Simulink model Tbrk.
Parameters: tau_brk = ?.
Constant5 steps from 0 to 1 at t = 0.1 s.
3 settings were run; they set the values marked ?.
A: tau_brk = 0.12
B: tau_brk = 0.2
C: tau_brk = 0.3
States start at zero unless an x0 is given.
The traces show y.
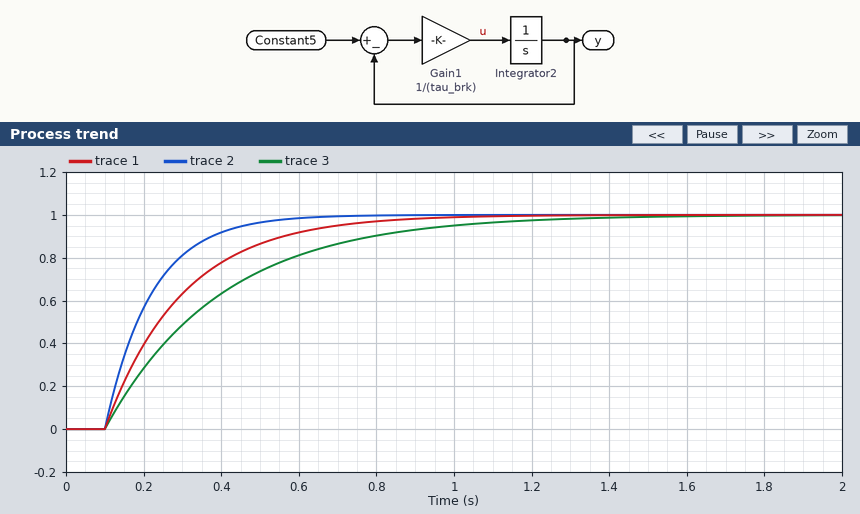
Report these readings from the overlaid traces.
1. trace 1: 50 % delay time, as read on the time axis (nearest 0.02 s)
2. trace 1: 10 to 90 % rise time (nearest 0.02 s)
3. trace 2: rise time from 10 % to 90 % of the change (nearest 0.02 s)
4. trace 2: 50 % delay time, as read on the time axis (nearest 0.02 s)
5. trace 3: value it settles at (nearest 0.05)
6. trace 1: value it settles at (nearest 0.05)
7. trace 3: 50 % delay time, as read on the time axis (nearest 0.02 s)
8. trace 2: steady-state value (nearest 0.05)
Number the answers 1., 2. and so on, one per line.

1. 0.24 s
2. 0.44 s
3. 0.26 s
4. 0.18 s
5. 1.00
6. 1.00
7. 0.30 s
8. 1.00
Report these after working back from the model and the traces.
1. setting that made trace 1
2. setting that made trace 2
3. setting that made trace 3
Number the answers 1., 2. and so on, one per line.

1. B
2. A
3. C
